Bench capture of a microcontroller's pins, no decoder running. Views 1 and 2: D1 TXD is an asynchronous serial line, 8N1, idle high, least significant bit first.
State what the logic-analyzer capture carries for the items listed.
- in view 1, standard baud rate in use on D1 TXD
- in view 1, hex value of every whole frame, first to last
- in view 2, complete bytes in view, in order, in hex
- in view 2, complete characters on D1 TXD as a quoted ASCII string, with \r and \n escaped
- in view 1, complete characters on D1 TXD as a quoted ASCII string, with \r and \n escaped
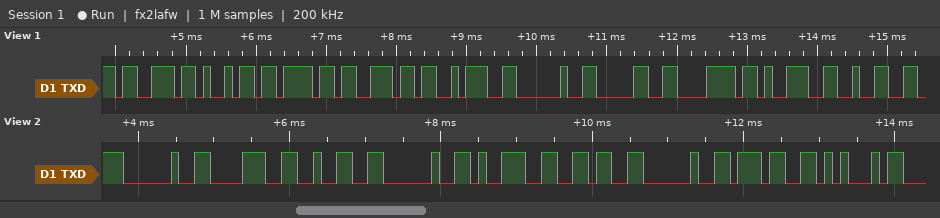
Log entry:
9600 baud
0x73 0x69 0x6F 0x6E 0x3A 0x20 0x30 0x78 0x39 0x32
20 38 32 20 39 36 20 37 45
" 82 96 7E"
"sion: 0x92"
